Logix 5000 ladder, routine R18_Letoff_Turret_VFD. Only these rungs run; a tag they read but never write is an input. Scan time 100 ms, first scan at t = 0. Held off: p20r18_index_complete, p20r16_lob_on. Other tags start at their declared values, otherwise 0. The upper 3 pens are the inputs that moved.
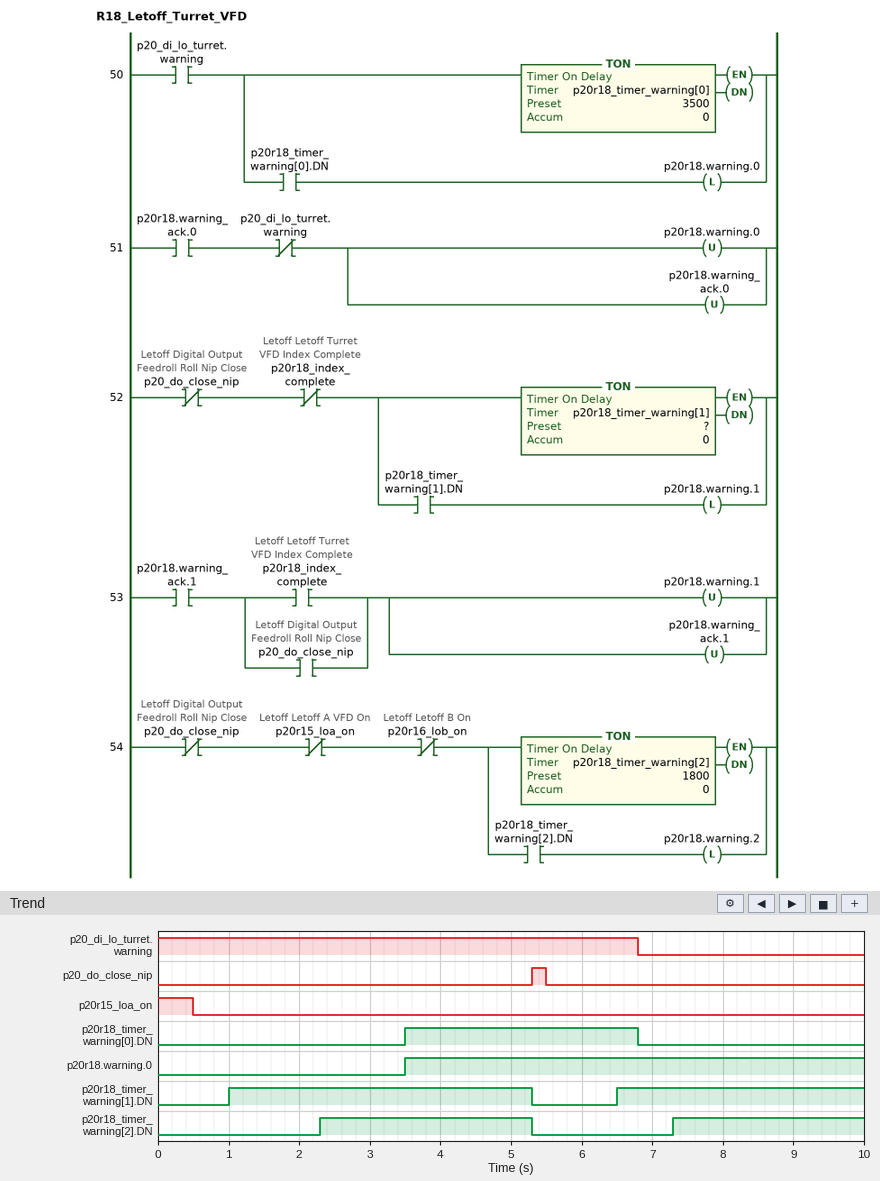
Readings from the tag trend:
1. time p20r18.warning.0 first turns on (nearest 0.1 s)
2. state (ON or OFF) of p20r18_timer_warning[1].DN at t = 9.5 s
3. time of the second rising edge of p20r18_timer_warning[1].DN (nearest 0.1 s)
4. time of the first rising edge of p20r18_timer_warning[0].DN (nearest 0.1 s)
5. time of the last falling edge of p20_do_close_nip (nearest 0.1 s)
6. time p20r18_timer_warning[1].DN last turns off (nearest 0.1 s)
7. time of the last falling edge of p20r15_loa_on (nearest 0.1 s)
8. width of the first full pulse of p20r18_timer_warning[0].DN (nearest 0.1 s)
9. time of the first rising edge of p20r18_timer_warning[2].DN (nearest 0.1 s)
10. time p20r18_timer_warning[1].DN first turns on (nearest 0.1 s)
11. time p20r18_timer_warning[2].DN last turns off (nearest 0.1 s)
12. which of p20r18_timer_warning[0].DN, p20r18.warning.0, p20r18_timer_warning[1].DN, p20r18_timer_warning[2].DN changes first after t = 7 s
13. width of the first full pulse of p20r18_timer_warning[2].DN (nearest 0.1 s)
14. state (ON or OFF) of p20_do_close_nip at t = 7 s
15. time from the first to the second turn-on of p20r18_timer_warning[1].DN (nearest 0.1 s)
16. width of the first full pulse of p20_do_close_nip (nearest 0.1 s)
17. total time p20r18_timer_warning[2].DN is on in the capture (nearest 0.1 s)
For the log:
3.5 s
ON
6.5 s
3.5 s
5.5 s
5.3 s
0.5 s
3.3 s
2.3 s
1.0 s
5.3 s
p20r18_timer_warning[2].DN
3.0 s
OFF
5.5 s
0.2 s
5.7 s
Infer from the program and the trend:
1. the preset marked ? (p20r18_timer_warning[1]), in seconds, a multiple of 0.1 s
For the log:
1.0 s
